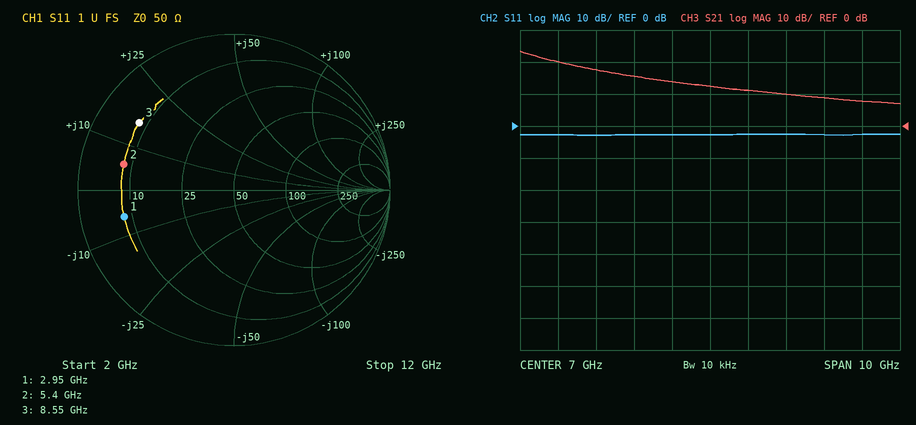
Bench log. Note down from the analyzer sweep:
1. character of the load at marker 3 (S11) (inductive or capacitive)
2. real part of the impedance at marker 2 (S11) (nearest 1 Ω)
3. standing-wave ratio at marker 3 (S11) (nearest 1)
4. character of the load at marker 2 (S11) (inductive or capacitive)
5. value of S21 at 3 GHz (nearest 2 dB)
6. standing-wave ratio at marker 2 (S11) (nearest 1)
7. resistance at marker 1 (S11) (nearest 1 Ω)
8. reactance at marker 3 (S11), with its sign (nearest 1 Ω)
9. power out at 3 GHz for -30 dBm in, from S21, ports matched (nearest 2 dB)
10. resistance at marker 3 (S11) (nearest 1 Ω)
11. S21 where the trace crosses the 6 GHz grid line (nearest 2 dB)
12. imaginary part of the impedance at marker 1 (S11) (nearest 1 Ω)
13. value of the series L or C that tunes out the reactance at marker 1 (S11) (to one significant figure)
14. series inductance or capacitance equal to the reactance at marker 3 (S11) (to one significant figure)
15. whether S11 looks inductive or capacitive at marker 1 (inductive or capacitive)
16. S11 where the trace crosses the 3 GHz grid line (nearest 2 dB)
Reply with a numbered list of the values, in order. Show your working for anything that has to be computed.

1. inductive
2. 8 Ω
3. 7
4. inductive
5. 20 dB
6. 6
7. 8 Ω
8. +16 Ω
9. -30 dBm + (20 dB) = -10 dBm
10. 8 Ω
11. 14 dB
12. -6 Ω
13. L = 6 Ω/(2π × 2.95 GHz) ≈ 324 pH, so 300 pH to one significant figure
14. L = 16 Ω/(2π × 8.55 GHz) ≈ 298 pH, so 300 pH to one significant figure
15. capacitive
16. -2 dB
